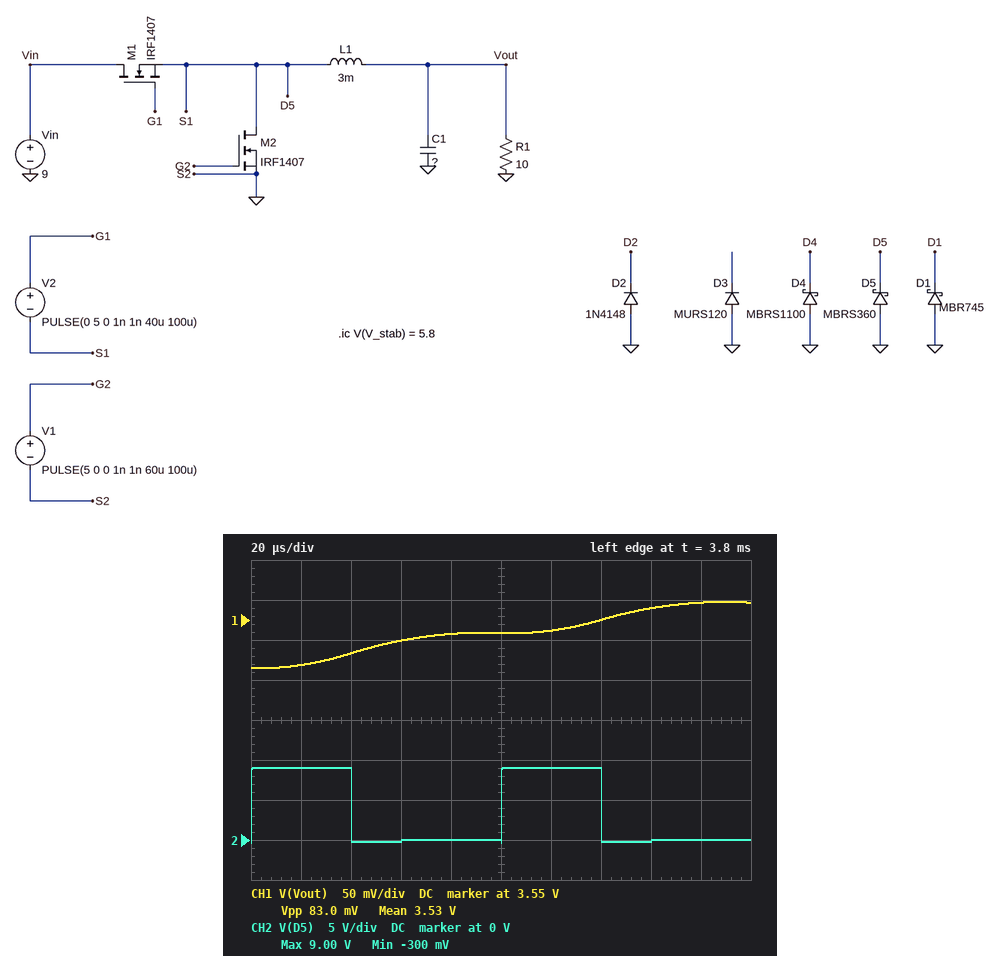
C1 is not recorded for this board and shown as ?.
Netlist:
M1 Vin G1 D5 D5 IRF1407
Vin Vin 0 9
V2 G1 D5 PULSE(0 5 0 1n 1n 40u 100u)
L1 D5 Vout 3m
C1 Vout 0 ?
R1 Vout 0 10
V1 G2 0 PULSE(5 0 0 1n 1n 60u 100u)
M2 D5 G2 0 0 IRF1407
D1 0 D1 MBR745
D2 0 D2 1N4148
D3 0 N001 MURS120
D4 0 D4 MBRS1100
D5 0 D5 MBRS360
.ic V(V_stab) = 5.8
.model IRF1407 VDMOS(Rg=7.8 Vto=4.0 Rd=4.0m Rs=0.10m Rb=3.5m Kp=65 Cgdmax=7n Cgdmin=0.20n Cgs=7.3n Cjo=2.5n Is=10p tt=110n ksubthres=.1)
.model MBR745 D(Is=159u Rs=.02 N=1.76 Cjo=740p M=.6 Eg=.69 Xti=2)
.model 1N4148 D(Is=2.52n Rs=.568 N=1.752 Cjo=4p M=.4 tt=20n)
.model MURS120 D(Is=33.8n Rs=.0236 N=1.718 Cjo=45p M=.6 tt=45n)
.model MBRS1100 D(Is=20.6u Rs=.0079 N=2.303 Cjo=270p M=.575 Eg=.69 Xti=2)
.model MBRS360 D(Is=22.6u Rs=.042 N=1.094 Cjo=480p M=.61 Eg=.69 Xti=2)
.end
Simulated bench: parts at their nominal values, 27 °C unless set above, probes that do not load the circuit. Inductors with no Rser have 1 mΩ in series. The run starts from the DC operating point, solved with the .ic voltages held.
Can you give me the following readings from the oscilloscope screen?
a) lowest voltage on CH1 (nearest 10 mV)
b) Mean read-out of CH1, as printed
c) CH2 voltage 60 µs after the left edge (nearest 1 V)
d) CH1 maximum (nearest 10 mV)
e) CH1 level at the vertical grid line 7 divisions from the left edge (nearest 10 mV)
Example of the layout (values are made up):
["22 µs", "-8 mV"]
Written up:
["3.49 V", "3.53 V", "0 V", "3.57 V", "3.55 V"]
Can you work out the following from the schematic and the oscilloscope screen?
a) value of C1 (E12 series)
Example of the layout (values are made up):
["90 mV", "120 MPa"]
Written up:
["68 µF"]
